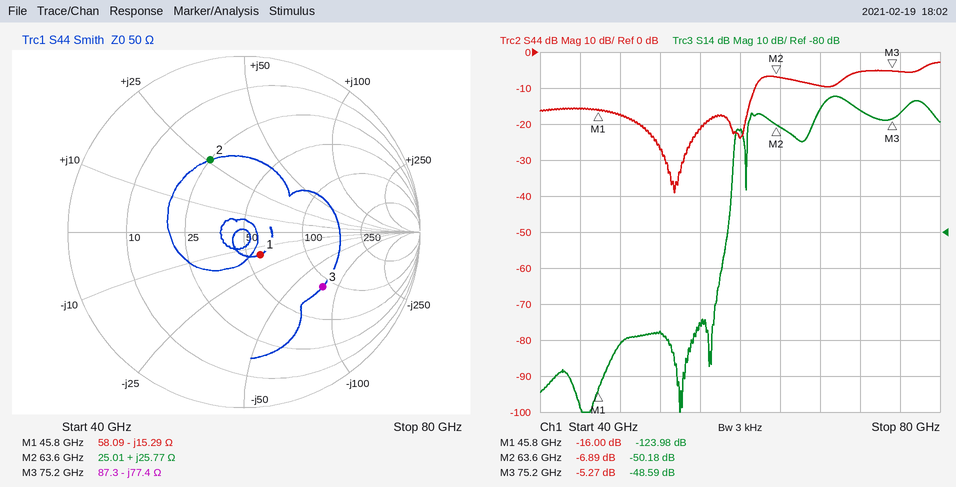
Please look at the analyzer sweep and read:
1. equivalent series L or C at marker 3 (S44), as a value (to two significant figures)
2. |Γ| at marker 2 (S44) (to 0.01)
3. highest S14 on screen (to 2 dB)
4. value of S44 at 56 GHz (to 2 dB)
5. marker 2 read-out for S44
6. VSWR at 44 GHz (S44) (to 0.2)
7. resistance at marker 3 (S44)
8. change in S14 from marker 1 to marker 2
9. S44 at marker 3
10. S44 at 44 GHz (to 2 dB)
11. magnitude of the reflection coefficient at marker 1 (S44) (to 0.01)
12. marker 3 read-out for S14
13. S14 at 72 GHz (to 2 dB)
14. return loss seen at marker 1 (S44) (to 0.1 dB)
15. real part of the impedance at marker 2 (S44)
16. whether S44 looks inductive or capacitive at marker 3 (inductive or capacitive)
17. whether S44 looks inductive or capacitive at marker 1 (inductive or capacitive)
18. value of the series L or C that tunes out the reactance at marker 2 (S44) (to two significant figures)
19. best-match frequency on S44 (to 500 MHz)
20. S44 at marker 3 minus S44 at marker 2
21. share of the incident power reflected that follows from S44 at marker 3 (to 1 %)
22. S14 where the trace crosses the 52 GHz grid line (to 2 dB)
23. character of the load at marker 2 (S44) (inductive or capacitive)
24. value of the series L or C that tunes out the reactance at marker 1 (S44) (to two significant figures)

27 fF
0.45
-42 dB
-22 dB
-6.89 dB
1.4
87.3 Ω
73.80 dB
-5.27 dB
-16 dB
0.16
-48.59 dB
-46 dB
16.0 dB
25.01 Ω
capacitive
capacitive
97 fF
53.5 GHz
1.62 dB
30 %
-108 dB
inductive
53 pH
